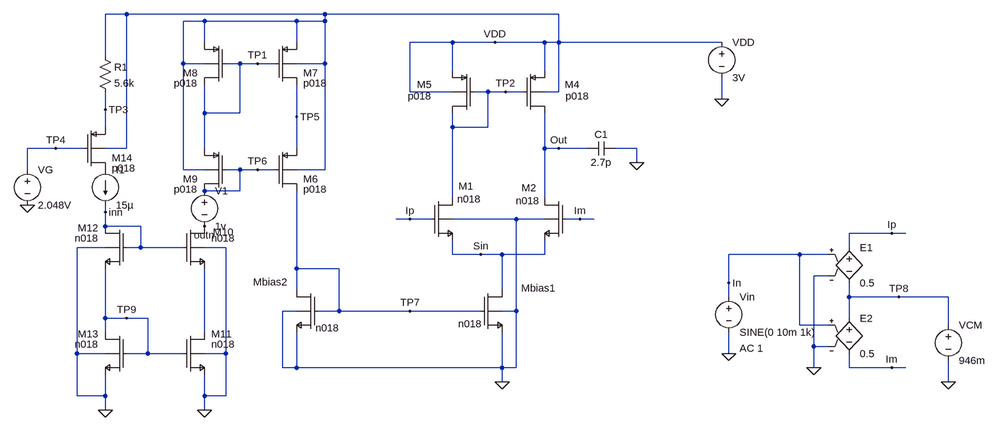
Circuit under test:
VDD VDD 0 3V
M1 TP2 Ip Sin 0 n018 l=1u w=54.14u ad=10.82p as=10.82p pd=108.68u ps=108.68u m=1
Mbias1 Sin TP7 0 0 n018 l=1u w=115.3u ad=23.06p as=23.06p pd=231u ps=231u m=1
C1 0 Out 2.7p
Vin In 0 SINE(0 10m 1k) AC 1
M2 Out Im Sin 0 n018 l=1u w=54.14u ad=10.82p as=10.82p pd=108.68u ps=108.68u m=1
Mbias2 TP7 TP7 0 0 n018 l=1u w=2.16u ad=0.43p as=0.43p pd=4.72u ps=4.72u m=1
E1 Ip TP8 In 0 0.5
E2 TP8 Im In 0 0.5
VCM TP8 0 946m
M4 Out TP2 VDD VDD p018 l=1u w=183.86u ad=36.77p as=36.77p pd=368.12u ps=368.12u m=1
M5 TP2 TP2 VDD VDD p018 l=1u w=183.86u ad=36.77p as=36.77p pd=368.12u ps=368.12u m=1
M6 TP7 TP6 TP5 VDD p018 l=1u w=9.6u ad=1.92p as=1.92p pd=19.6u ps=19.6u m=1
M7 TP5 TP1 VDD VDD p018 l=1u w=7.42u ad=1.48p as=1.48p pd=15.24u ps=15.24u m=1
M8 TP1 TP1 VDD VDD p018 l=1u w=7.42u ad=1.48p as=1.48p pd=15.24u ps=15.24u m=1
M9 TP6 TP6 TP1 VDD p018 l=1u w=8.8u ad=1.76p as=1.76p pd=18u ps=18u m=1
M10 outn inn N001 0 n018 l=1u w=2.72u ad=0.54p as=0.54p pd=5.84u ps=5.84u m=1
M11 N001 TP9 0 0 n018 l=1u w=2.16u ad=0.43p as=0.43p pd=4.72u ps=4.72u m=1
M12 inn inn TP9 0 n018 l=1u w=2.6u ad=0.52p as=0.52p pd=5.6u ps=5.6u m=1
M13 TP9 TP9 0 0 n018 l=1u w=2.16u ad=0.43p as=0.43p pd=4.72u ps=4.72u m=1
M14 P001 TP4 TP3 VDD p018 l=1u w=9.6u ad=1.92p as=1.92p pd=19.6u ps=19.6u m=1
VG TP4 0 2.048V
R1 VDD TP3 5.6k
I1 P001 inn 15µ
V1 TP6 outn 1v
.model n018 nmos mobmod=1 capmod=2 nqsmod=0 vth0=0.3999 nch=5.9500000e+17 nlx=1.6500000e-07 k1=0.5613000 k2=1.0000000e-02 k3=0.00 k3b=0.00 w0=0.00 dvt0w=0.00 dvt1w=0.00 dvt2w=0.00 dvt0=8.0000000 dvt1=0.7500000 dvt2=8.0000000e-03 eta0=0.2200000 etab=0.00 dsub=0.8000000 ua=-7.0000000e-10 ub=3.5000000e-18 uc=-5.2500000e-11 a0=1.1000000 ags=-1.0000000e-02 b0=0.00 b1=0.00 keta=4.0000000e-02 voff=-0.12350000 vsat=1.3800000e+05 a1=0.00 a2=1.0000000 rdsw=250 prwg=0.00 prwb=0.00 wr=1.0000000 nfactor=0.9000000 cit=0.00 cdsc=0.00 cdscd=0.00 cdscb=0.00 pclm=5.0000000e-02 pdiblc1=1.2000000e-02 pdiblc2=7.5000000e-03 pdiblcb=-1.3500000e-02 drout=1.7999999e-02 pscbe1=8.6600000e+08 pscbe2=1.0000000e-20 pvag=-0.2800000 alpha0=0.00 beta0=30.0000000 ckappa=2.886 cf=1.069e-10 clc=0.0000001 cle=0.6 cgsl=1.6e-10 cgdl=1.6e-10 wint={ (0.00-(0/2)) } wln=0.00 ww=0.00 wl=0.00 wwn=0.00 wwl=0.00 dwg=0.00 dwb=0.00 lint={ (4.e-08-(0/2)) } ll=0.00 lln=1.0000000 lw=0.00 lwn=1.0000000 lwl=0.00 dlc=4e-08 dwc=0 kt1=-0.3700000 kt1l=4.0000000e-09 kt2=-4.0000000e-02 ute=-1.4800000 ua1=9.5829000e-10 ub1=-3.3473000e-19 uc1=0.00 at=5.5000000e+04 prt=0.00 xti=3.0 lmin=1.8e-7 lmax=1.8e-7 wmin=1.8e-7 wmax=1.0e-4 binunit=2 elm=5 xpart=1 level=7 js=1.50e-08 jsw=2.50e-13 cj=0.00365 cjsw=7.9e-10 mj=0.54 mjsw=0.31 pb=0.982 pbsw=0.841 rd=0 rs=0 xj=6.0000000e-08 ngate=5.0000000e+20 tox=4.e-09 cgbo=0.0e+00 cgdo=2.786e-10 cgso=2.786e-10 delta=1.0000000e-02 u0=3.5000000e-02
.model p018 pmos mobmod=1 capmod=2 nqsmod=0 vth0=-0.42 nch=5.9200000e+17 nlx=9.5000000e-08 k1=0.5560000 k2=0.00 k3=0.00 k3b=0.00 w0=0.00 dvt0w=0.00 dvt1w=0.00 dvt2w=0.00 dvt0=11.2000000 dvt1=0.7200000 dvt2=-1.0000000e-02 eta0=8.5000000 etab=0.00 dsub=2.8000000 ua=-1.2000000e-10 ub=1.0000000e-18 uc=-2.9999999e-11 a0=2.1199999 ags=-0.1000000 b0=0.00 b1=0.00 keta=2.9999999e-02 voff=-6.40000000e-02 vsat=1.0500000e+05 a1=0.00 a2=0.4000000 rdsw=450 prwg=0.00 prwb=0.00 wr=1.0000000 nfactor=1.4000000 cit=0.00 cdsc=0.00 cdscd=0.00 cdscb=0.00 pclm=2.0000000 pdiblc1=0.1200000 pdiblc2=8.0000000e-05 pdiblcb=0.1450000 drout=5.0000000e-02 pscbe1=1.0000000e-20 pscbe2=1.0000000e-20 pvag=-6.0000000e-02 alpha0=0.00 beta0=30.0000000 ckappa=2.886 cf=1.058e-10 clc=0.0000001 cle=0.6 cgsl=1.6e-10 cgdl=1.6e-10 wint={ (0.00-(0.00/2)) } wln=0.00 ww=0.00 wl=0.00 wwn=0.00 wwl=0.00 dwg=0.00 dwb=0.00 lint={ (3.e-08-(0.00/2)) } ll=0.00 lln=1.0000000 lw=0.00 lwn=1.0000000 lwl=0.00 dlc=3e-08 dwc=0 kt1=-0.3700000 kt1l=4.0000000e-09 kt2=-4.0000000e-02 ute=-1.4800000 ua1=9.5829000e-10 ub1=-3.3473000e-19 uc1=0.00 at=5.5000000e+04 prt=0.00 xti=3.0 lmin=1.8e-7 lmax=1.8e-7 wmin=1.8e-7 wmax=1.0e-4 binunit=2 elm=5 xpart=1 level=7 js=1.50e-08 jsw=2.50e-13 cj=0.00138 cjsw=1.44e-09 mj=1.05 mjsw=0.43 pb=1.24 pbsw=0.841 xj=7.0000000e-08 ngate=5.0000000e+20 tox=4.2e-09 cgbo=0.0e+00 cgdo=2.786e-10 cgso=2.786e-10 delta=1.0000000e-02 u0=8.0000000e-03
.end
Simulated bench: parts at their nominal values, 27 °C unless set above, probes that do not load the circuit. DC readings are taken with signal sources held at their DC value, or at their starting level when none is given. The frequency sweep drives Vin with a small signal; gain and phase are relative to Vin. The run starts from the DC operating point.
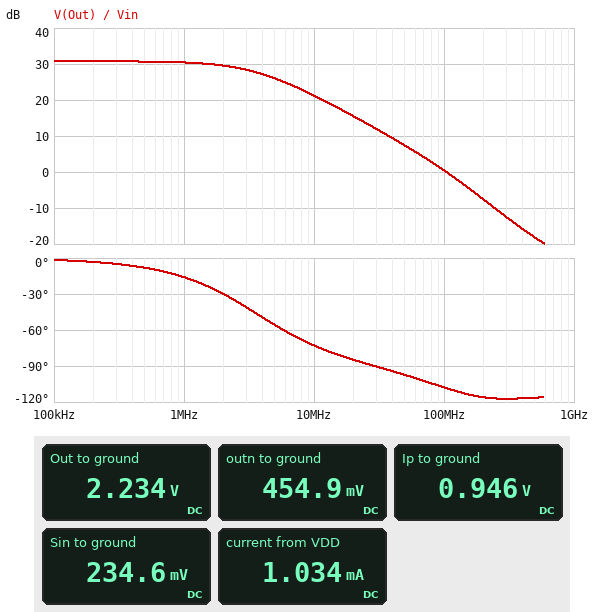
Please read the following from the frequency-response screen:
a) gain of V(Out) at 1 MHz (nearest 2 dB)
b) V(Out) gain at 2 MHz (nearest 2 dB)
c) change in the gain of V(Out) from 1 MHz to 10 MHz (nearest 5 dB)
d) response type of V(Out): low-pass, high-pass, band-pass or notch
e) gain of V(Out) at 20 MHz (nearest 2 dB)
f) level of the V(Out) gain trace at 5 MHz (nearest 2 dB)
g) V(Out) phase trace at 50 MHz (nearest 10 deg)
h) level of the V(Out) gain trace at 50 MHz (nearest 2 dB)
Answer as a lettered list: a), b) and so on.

a) 30 dB
b) 30 dB
c) -10 dB
d) low-pass
e) 16 dB
f) 26 dB
g) -100 deg
h) 8 dB
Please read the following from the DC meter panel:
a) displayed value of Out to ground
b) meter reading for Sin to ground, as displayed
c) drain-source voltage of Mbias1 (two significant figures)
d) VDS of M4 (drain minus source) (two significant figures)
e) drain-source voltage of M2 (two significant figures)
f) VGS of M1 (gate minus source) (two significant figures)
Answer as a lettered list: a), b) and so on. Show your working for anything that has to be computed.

a) 2.234 V
b) 234.6 mV
c) 234.6 mV = 230 mV
d) 2.234 V - 3 V = -770 mV
e) 2.234 V - 234.6 mV = 2.0 V
f) 946 mV - 234.6 mV = 710 mV
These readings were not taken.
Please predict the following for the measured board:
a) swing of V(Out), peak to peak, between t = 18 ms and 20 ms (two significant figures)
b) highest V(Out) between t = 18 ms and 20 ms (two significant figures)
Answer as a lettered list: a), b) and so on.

a) 840 mV
b) 2.5 V
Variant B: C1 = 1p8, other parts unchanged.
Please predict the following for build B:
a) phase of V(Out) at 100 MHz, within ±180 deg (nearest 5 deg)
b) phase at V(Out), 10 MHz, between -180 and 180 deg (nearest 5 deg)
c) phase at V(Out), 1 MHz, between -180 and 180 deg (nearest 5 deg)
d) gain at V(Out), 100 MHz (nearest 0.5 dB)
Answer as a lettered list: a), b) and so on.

a) -105 deg
b) -65 deg
c) -10 deg
d) 3.0 dB
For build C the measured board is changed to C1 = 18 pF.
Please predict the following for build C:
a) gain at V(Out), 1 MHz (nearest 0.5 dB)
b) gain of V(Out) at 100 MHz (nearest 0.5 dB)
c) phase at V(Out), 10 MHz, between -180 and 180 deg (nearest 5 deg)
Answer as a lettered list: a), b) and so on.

a) 25.5 dB
b) -14.5 dB
c) -90 deg
